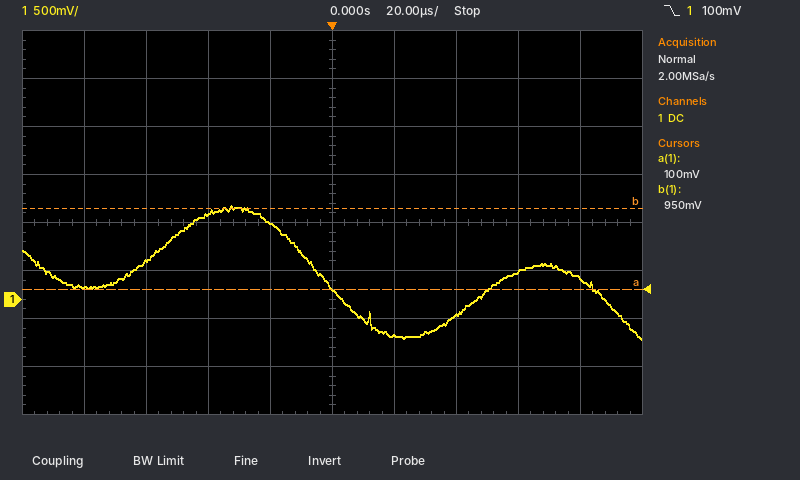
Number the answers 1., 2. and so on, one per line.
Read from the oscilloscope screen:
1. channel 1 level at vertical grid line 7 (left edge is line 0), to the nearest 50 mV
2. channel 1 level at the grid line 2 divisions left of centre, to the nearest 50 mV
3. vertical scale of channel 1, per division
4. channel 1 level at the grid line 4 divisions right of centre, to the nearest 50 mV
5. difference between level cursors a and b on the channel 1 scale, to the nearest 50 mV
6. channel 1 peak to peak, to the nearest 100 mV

1. -150 mV
2. 900 mV
3. 500 mV
4. 200 mV
5. 850 mV
6. 1.40 V
